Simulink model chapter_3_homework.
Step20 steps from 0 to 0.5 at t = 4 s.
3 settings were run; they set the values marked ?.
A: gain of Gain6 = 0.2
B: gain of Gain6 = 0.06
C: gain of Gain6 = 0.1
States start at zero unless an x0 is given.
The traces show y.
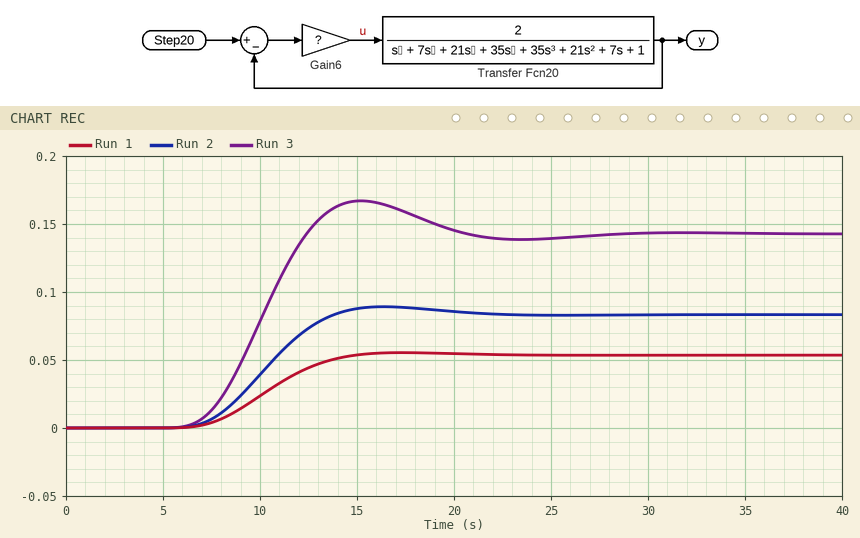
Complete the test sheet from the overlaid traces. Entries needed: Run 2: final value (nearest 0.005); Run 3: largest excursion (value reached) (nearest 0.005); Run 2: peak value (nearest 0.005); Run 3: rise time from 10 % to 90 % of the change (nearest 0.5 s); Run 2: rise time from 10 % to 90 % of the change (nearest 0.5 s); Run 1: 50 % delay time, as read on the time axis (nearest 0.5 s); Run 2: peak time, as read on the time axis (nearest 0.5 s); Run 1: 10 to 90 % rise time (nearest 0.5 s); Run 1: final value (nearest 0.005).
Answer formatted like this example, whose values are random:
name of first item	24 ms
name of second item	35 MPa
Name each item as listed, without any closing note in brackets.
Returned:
Run 2: final value	0.085
Run 3: largest excursion (value reached)	0.165
Run 2: peak value	0.090
Run 3: rise time from 10 % to 90 % of the change	4.0 s
Run 2: rise time from 10 % to 90 % of the change	5.0 s
Run 1: 50 % delay time, as read on the time axis	10.5 s
Run 2: peak time, as read on the time axis	16.5 s
Run 1: 10 to 90 % rise time	5.5 s
Run 1: final value	0.055
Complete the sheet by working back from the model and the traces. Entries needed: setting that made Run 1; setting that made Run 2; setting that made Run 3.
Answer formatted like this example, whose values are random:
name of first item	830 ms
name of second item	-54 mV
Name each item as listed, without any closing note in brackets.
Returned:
setting that made Run 1	B
setting that made Run 2	C
setting that made Run 3	A
